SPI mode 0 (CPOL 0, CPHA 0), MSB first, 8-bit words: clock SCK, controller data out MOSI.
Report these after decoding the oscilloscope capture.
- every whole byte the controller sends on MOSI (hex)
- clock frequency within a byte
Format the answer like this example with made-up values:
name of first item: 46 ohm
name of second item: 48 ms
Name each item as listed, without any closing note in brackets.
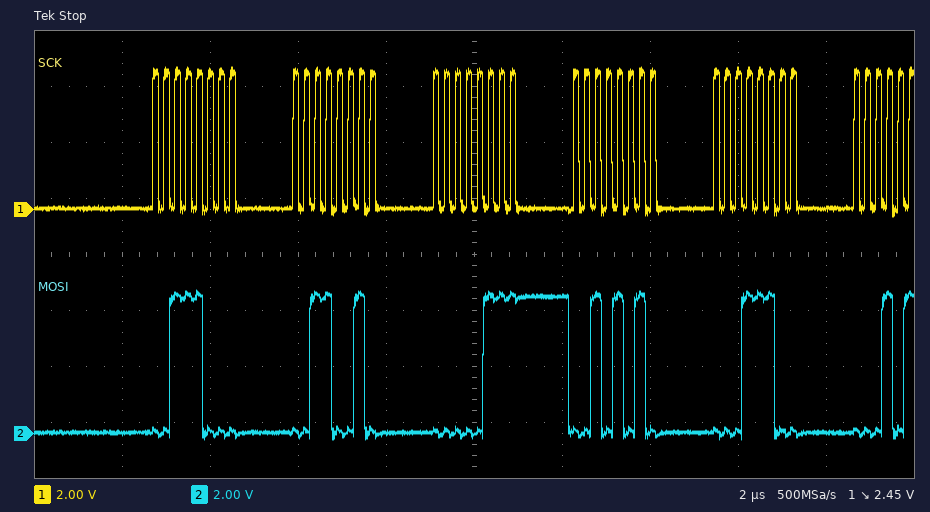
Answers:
every whole byte the controller sends on MOSI: 38 32 07 2A 1C
clock frequency within a byte: 4 MHz
